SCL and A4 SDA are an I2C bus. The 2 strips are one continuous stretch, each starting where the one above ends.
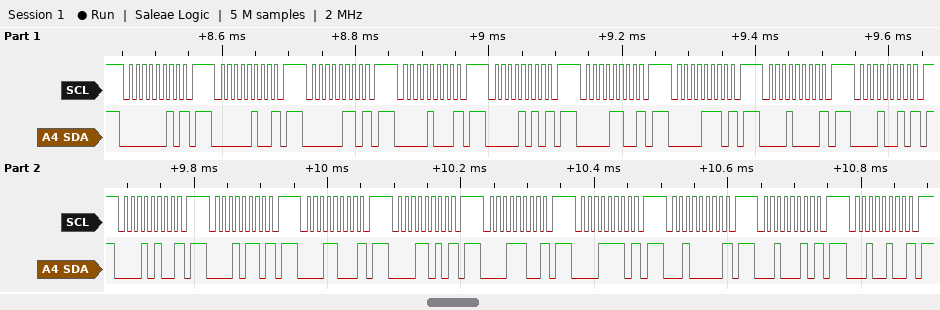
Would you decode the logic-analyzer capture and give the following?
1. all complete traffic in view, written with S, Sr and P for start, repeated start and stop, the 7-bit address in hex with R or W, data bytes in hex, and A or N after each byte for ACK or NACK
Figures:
S 01W N P S 02W N P S 03W N P S 04W N P S 05W N P S 06W N P S 07W N P S 08W N P S 09W N P S 0AW N P S 0BW N P S 0CW N P S 0DW N P S 0EW N P S 0FW N P S 10W N P S 11W N P S 12W N P
